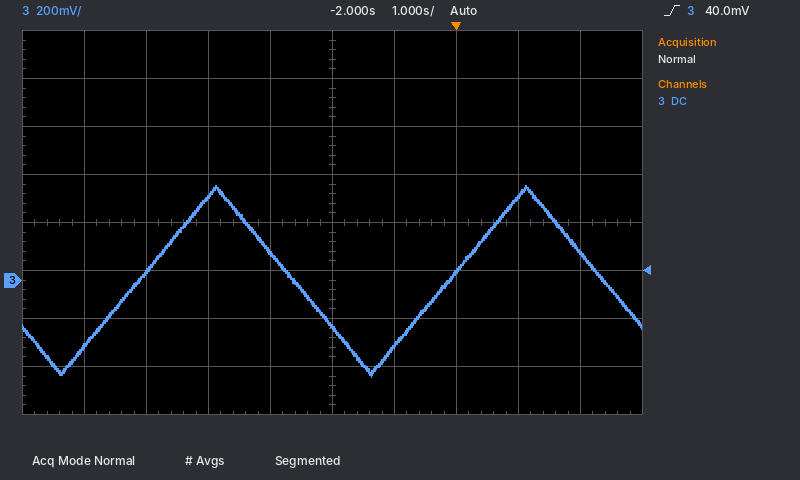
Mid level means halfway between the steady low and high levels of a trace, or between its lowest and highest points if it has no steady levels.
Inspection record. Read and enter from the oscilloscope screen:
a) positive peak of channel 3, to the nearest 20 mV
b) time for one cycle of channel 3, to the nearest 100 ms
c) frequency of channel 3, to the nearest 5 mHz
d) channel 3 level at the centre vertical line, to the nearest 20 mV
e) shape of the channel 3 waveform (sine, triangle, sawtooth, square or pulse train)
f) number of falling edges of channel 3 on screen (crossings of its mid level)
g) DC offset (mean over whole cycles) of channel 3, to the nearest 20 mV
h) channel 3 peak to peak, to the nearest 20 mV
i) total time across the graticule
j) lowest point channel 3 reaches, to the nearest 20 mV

400 mV
5.0 s
200 mHz
-200 mV
triangle
2
0 mV
800 mV
10 s
-400 mV
